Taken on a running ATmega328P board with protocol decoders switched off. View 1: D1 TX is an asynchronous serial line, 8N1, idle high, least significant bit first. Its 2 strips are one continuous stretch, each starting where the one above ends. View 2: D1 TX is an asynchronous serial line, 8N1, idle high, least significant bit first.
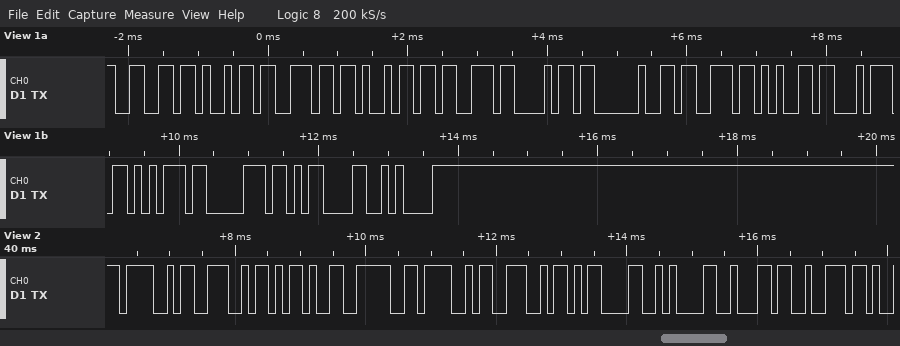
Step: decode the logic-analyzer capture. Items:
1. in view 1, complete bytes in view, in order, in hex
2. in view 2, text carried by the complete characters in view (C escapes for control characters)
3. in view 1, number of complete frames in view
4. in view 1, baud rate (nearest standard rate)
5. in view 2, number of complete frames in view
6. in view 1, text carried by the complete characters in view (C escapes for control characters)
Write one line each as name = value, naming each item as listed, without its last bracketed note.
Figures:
in view 1, complete bytes in view, in order, in hex = 66 69 6E 69 73 68 20 73 65 74 75 70 0D 0A
in view 2, text carried by the complete characters in view = "ON->ON\r\nbr"
in view 1, number of complete frames in view = 14
in view 1, baud rate = 9600 baud
in view 2, number of complete frames in view = 10
in view 1, text carried by the complete characters in view = "finish setup\r\n"
